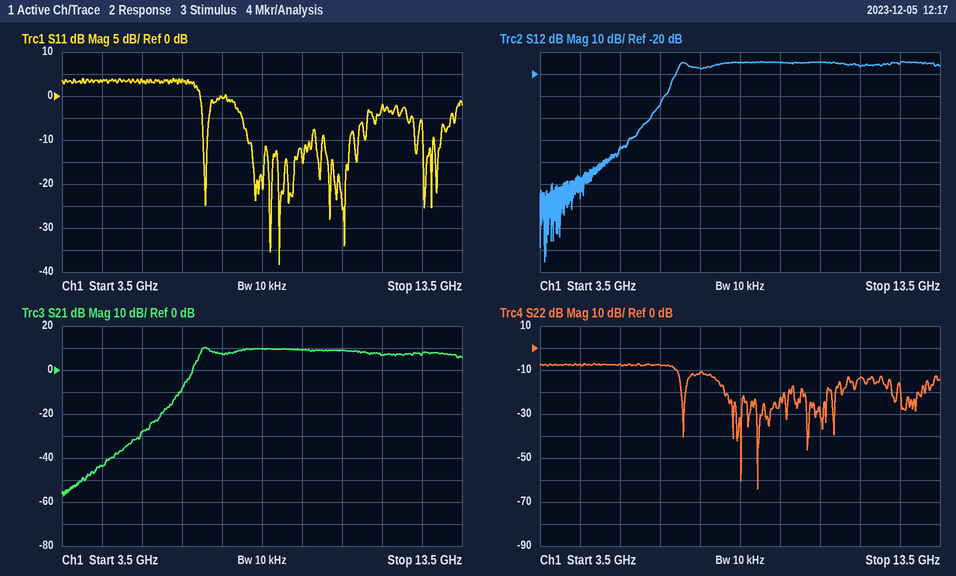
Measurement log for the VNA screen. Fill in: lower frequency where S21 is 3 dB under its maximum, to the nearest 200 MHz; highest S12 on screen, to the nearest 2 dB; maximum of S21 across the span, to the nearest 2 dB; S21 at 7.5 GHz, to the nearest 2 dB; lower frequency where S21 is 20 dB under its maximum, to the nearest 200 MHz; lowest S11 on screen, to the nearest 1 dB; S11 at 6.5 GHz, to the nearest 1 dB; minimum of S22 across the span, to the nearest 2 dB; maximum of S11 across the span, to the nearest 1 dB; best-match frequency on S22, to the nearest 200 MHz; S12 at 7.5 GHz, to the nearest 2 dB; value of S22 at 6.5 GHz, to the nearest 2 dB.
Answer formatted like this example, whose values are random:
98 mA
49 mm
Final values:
7.0 GHz
-14 dB
10 dB
8 dB
6.4 GHz
-38 dB
4 dB
-64 dB
4 dB
9.0 GHz
-18 dB
-8 dB
